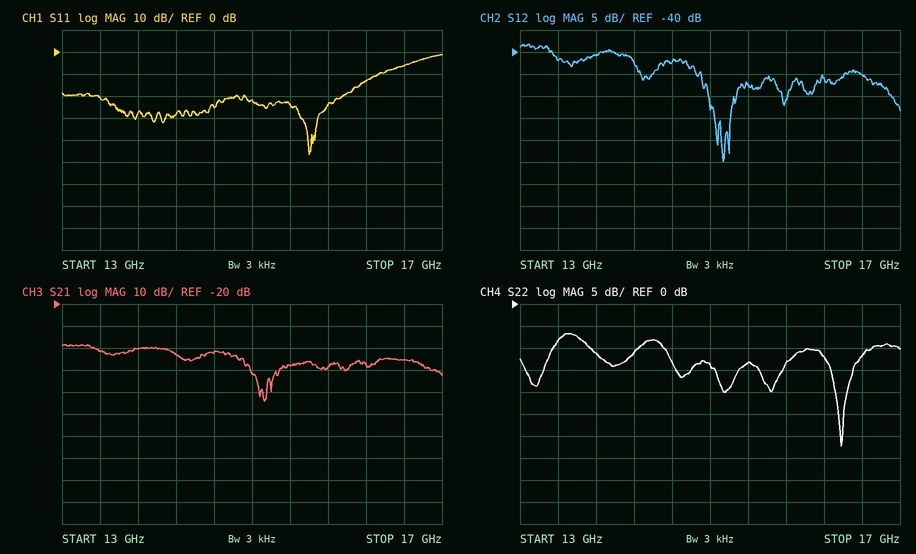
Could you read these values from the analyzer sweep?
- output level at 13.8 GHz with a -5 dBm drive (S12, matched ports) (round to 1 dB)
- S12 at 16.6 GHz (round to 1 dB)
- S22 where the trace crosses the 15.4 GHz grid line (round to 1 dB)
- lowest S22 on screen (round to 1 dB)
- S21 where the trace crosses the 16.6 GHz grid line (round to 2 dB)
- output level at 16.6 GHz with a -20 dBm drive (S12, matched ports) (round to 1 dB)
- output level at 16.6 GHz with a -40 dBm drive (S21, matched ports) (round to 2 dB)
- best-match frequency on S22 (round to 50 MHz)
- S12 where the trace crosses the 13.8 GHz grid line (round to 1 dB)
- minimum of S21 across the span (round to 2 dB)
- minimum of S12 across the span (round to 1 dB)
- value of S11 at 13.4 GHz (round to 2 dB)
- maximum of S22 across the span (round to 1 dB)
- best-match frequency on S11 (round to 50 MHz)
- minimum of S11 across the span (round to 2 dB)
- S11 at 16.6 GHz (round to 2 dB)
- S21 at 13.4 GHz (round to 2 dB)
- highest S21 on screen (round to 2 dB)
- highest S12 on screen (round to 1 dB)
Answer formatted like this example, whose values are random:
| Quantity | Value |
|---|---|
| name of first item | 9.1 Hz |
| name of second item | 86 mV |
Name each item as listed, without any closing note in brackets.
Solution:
| Quantity | Value |
|---|---|
| output level at 13.8 GHz with a -5 dBm drive (S12, matched ports) | -46 dBm |
| S12 at 16.6 GHz | -45 dB |
| S22 where the trace crosses the 15.4 GHz grid line | -13 dB |
| lowest S22 on screen | -32 dB |
| S21 where the trace crosses the 16.6 GHz grid line | -46 dB |
| output level at 16.6 GHz with a -20 dBm drive (S12, matched ports) | -65 dBm |
| output level at 16.6 GHz with a -40 dBm drive (S21, matched ports) | -86 dBm |
| best-match frequency on S22 | 16.40 GHz |
| S12 where the trace crosses the 13.8 GHz grid line | -41 dB |
| minimum of S21 across the span | -64 dB |
| minimum of S12 across the span | -65 dB |
| value of S11 at 13.4 GHz | -20 dB |
| maximum of S22 across the span | -7 dB |
| best-match frequency on S11 | 15.60 GHz |
| minimum of S11 across the span | -46 dB |
| S11 at 16.6 GHz | -6 dB |
| S21 at 13.4 GHz | -42 dB |
| highest S21 on screen | -38 dB |
| highest S12 on screen | -38 dB |
